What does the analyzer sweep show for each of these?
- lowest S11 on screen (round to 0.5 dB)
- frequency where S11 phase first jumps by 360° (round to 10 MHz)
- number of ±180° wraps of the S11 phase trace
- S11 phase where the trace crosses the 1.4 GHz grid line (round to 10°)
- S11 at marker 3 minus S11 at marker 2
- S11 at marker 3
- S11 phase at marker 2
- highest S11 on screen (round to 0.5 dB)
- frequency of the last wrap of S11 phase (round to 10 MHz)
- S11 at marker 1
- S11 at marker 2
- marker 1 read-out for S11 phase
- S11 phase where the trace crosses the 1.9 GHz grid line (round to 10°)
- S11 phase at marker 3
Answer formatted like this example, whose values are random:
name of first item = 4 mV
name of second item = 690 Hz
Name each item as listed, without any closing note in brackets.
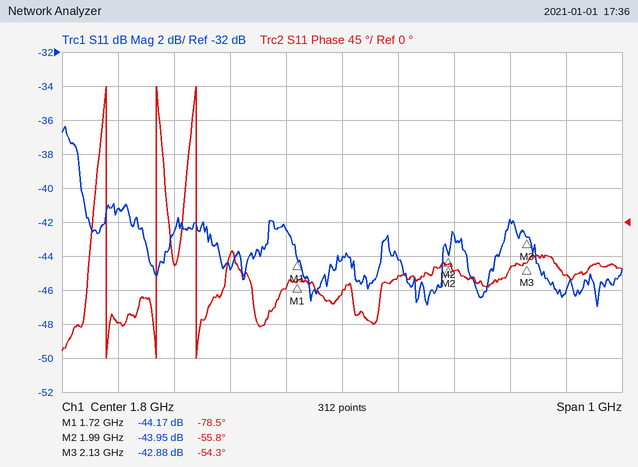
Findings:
lowest S11 on screen = -47.0 dB
frequency where S11 phase first jumps by 360° = 1.38 GHz
number of ±180° wraps of the S11 phase trace = 3
S11 phase where the trace crosses the 1.4 GHz grid line = -130°
S11 at marker 3 minus S11 at marker 2 = 1.07 dB
S11 at marker 3 = -42.88 dB
S11 phase at marker 2 = -55.8°
highest S11 on screen = -36.5 dB
frequency of the last wrap of S11 phase = 1.54 GHz
S11 at marker 1 = -44.17 dB
S11 at marker 2 = -43.95 dB
marker 1 read-out for S11 phase = -78.5°
S11 phase where the trace crosses the 1.9 GHz grid line = -70°
S11 phase at marker 3 = -54.3°
